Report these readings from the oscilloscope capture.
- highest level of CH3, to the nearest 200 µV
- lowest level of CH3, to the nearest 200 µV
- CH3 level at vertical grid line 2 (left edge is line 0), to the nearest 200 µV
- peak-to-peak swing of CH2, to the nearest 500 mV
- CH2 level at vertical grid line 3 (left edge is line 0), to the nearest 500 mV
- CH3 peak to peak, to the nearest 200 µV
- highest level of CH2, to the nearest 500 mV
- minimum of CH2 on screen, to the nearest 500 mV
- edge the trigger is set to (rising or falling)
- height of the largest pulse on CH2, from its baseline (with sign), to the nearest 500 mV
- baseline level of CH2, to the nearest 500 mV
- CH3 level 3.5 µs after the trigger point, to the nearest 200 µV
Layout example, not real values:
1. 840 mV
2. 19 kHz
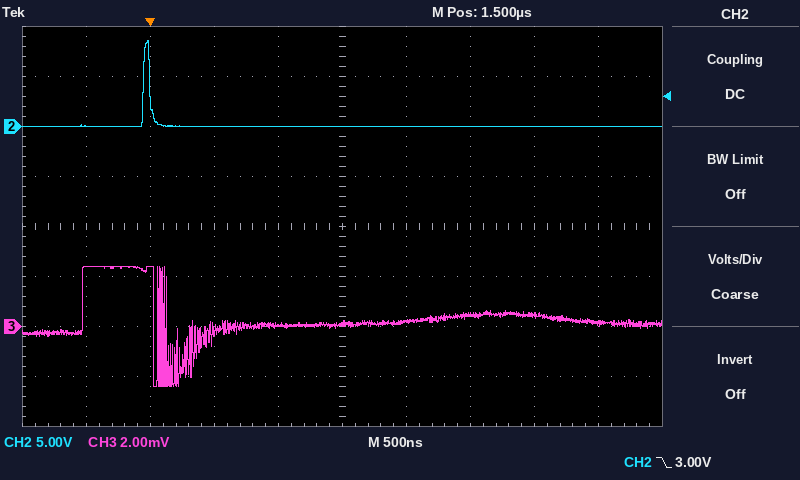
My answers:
1. 2.4 mV
2. -2.4 mV
3. 2.4 mV
4. 8.5 V
5. 0.0 V
6. 4.8 mV
7. 8.5 V
8. 0.0 V
9. falling
10. +8.5 V
11. 0.0 V
12. 200 µV
